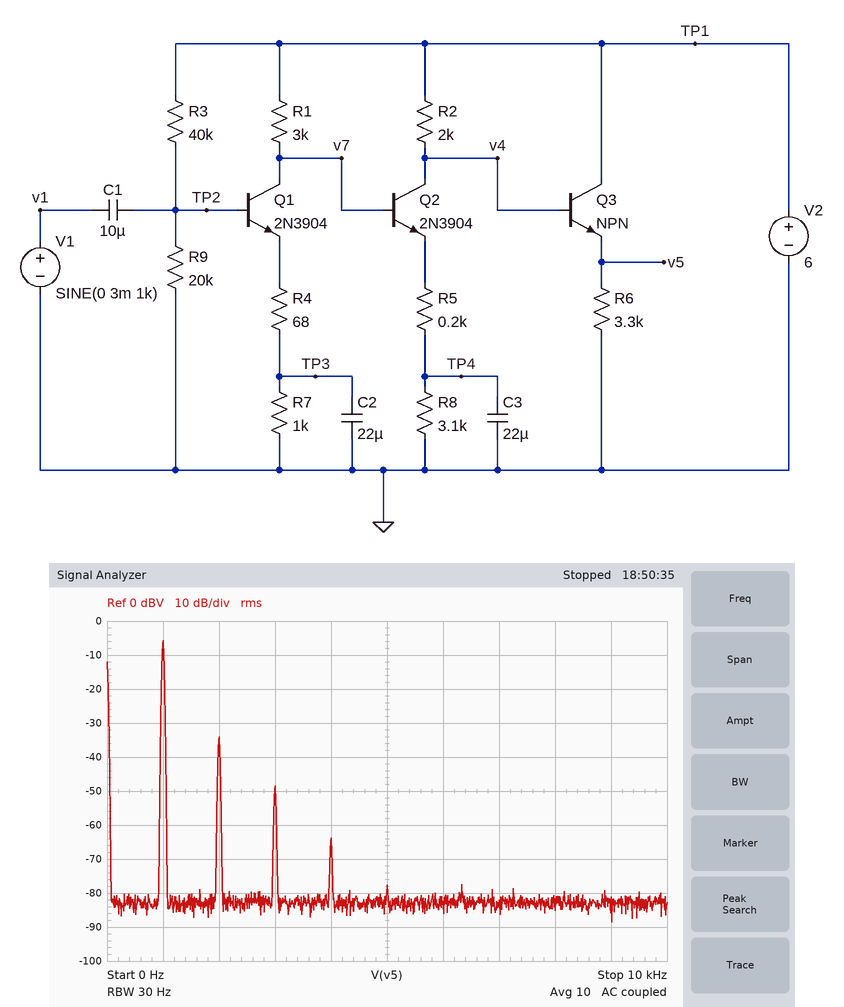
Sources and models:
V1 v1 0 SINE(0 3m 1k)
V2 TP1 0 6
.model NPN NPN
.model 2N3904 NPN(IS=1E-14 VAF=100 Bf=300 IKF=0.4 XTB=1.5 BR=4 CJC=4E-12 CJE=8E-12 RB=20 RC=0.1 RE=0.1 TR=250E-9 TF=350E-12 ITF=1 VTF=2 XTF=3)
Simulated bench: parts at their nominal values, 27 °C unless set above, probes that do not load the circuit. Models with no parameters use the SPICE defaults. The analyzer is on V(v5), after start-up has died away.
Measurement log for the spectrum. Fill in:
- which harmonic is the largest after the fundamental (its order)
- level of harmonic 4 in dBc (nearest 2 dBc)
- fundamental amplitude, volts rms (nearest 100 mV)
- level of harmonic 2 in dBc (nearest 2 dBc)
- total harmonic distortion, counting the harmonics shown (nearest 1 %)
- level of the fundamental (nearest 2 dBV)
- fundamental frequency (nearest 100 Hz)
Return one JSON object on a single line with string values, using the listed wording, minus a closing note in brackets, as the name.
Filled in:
{"which harmonic is the largest after the fundamental": "2", "level of harmonic 4 in dBc": "-58 dBc", "fundamental amplitude, volts rms": "500 mV", "level of harmonic 2 in dBc": "-28 dBc", "total harmonic distortion, counting the harmonics shown": "4 %", "level of the fundamental": "-6 dBV", "fundamental frequency": "1.0 kHz"}
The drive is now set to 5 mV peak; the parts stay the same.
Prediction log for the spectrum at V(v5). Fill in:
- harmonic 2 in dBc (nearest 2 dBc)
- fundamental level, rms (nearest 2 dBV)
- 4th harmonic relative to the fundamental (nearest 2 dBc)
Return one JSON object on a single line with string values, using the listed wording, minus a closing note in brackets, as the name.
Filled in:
{"harmonic 2 in dBc": "-20 dBc", "fundamental level, rms": "-2 dBV", "4th harmonic relative to the fundamental": "-44 dBc"}
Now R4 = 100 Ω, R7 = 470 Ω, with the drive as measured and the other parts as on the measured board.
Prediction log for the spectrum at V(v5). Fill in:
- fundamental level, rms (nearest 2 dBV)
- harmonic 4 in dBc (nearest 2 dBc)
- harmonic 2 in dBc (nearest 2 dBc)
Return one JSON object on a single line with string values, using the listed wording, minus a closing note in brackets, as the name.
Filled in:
{"fundamental level, rms": "-26 dBV", "harmonic 4 in dBc": "-48 dBc", "harmonic 2 in dBc": "-16 dBc"}
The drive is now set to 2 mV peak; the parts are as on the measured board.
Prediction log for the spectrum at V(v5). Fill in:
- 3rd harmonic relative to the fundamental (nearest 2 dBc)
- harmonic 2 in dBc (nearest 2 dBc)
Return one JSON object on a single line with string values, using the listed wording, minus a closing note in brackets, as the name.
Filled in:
{"3rd harmonic relative to the fundamental": "-50 dBc", "harmonic 2 in dBc": "-32 dBc"}
